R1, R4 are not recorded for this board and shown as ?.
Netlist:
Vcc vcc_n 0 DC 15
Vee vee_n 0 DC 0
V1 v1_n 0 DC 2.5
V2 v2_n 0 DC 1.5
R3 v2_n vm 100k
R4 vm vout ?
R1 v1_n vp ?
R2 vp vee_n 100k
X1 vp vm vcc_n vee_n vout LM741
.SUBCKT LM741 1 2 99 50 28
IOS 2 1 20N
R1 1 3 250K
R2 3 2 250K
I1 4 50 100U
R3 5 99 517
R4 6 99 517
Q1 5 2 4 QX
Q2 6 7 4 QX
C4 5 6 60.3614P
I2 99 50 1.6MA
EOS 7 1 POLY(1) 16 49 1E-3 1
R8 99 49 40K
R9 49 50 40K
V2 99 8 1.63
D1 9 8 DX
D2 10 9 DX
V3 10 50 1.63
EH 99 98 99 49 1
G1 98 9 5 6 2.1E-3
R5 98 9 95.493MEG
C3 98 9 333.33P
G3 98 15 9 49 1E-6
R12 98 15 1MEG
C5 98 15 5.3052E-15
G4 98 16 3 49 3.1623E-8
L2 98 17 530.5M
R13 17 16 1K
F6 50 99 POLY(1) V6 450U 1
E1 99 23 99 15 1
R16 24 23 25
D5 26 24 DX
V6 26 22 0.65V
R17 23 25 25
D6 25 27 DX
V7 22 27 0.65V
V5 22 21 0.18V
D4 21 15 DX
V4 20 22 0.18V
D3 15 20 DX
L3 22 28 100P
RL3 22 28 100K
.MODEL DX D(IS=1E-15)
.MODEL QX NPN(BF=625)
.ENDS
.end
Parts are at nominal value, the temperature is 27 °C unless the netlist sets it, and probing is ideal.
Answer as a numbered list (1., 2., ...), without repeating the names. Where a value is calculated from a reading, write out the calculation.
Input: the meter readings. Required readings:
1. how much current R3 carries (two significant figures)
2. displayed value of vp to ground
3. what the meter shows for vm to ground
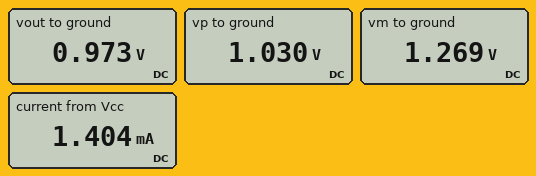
1. (1.5 V - 1.269 V) / 100 kΩ = 2.3 µA
2. 1.030 V
3. 1.269 V
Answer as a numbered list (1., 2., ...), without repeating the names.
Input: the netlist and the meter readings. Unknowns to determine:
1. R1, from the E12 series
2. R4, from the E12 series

1. 150 kΩ
2. 180 kΩ
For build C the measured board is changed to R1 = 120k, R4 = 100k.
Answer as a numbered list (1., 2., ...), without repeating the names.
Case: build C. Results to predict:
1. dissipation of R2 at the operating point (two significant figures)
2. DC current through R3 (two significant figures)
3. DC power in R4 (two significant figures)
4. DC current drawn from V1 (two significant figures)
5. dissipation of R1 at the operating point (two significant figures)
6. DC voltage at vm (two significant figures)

1. 13 µW
2. 2.8 µA
3. 600 nW
4. 11 µA
5. 15 µW
6. 1.2 V
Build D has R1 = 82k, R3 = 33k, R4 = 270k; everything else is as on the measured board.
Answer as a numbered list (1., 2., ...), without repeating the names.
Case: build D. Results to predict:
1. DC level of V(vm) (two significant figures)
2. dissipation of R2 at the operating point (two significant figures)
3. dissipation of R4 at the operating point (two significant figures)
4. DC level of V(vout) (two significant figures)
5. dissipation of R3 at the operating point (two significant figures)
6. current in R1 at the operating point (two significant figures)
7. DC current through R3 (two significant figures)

1. 1.4 V
2. 19 µW
3. 770 nW
4. 980 mV
5. 130 nW
6. 14 µA
7. 2.0 µA
